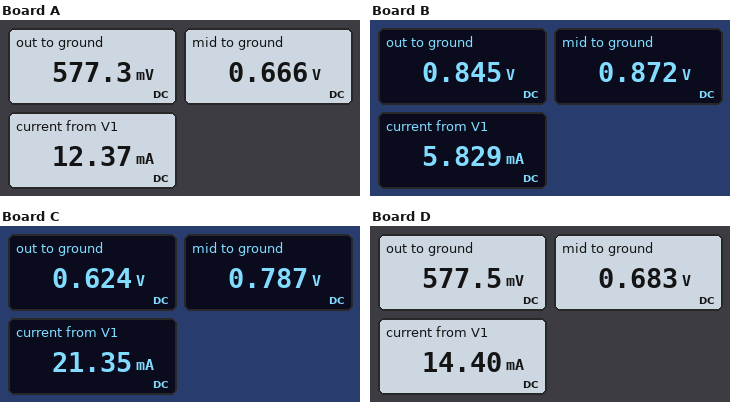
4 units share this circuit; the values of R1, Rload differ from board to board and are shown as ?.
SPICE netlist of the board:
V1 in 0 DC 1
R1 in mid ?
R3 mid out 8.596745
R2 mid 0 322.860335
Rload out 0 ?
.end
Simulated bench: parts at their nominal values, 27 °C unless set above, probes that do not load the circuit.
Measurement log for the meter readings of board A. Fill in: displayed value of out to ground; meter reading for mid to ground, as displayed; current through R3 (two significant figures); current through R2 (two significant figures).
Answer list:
577.3 mV
0.666 V
10 mA
2.1 mA
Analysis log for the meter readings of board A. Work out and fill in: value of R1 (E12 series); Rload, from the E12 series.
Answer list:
27 Ω
56 Ω
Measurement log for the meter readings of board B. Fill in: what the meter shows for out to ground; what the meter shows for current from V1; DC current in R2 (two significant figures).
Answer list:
0.845 V
5.829 mA
2.7 mA
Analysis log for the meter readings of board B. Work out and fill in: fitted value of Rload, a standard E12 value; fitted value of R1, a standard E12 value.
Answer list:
270 Ω
22 Ω
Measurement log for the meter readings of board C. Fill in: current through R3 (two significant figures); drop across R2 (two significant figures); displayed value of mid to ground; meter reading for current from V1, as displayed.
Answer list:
19 mA
790 mV
0.787 V
21.35 mA
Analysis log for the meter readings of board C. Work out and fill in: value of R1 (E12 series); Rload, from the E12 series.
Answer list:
10 Ω
33 Ω
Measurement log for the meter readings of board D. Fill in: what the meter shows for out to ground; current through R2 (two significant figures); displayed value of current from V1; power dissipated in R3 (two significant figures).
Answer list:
577.5 mV
2.1 mA
14.40 mA
1.3 mW
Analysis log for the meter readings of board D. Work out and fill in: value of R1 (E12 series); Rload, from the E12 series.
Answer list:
22 Ω
47 Ω
